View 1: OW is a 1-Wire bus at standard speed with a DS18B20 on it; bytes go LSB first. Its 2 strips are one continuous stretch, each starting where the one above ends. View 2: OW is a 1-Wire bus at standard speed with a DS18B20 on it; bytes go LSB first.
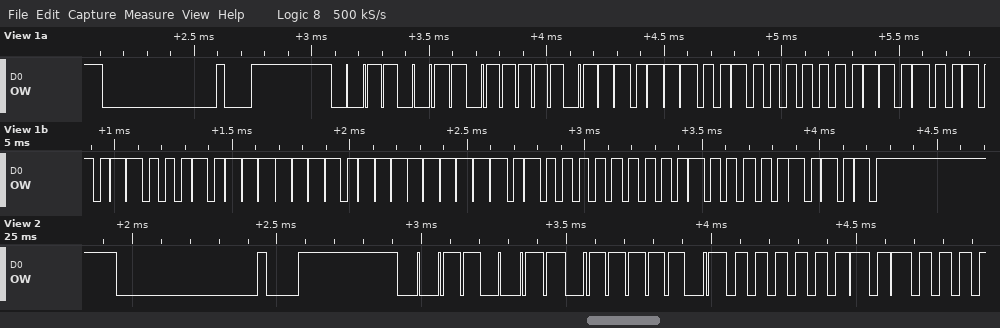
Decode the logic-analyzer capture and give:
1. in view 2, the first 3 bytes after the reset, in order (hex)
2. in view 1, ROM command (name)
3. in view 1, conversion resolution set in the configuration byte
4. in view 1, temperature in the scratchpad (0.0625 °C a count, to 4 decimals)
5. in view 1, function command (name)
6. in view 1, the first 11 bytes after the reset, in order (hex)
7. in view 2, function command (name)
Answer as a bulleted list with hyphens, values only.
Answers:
- CC BE 40
- Skip ROM
- 12 bits
- 19.6875 °C
- Read Scratchpad
- CC BE 3B 01 4B 46 7F FF 05 10 54
- Read Scratchpad
